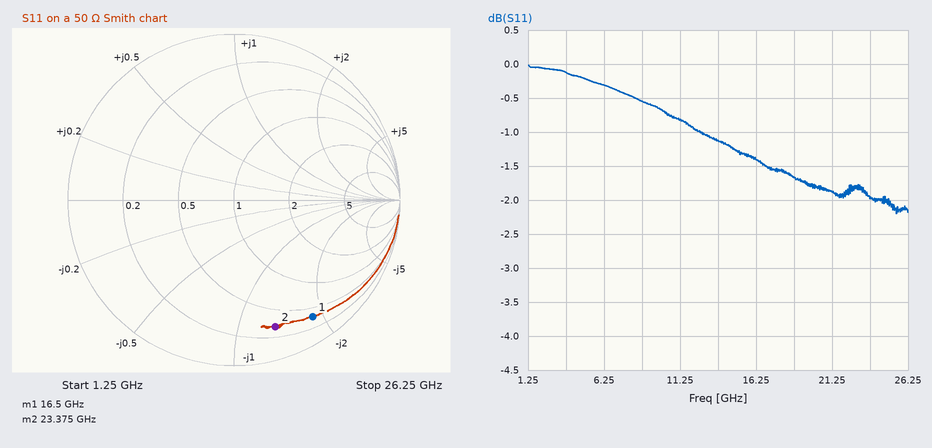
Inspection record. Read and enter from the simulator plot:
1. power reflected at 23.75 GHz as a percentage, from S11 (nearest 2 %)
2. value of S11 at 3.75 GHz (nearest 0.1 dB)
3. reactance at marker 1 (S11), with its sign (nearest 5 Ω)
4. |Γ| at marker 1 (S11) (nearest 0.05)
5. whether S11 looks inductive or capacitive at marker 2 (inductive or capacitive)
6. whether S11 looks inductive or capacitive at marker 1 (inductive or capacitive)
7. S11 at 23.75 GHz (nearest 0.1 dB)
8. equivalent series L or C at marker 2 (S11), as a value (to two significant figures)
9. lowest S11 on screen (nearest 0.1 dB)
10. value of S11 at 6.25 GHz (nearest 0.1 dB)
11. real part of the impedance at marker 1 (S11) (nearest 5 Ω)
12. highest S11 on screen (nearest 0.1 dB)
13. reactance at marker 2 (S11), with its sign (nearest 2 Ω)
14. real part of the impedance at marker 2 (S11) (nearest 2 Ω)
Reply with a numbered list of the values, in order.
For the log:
1. 64 %
2. -0.1 dB
3. -90 Ω
4. 0.85
5. capacitive
6. capacitive
7. -2.0 dB
8. 100 fF
9. -2.2 dB
10. -0.3 dB
11. 20 Ω
12. 0.0 dB
13. -66 Ω
14. 16 Ω
